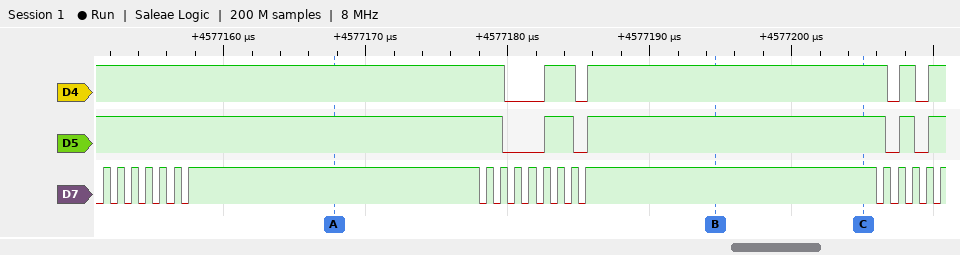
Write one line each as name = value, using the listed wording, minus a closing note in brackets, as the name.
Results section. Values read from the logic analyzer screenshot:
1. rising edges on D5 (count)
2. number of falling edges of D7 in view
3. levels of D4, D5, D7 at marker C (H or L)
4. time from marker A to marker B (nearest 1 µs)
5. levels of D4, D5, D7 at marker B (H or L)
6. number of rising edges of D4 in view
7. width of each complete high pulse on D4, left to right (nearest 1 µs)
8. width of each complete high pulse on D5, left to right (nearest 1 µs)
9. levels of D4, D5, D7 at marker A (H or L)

rising edges on D5 = 4
number of falling edges of D7 in view = 19
levels of D4, D5, D7 at marker C = D4=H, D5=H, D7=H
time from marker A to marker B = 27 µs
levels of D4, D5, D7 at marker B = D4=H, D5=H, D7=H
number of rising edges of D4 in view = 4
width of each complete high pulse on D4, left to right = 2 µs, 21 µs, 1 µs
width of each complete high pulse on D5, left to right = 2 µs, 21 µs, 1 µs
levels of D4, D5, D7 at marker A = D4=H, D5=H, D7=H
